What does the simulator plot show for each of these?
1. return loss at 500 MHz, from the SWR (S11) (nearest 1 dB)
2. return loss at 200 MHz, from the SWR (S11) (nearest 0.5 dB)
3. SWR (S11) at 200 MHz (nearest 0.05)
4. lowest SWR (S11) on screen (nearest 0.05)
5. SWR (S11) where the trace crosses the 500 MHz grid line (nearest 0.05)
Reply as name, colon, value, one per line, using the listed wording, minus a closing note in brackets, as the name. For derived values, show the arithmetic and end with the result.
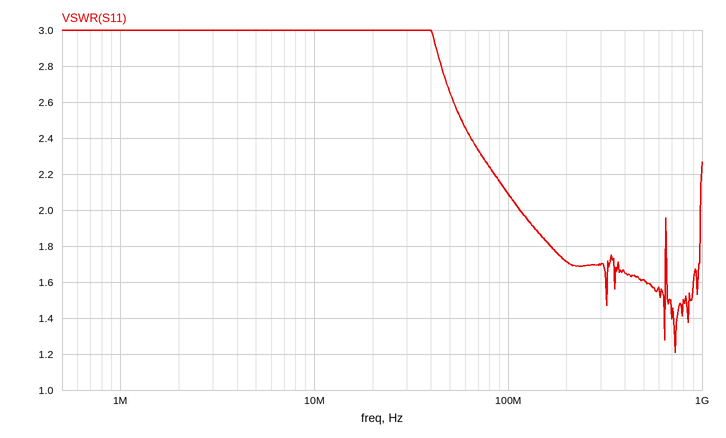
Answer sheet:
return loss at 500 MHz, from the SWR (S11): −20 log10((1.6 − 1)/(1.6 + 1)) ≈ 13 dB
return loss at 200 MHz, from the SWR (S11): −20 log10((1.7 − 1)/(1.7 + 1)) ≈ 11.7 dB, so 11.5 dB to the nearest 0.5 dB
SWR (S11) at 200 MHz: 1.70
lowest SWR (S11) on screen: 1.20
SWR (S11) where the trace crosses the 500 MHz grid line: 1.60
